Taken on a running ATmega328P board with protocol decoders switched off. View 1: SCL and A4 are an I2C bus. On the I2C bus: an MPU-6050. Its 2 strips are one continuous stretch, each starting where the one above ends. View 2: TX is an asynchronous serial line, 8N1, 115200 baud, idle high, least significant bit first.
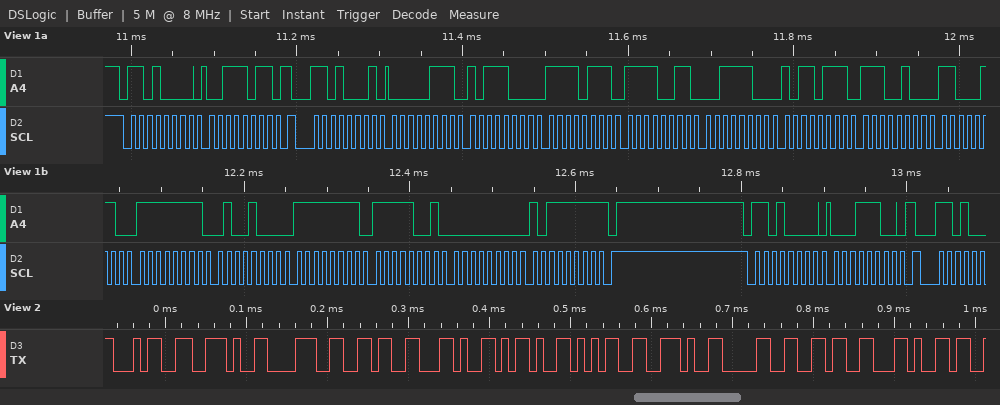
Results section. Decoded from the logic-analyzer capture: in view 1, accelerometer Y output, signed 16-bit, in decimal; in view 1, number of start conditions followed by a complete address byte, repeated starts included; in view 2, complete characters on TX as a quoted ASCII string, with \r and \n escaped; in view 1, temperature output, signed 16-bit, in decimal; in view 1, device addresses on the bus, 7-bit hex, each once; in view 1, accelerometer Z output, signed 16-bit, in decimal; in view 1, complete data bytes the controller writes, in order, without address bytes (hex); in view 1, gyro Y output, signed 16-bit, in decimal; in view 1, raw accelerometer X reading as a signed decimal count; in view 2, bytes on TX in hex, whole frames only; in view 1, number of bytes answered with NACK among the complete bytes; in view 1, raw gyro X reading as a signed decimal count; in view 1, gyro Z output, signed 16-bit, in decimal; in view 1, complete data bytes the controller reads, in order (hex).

-2061
3
"4.86,-5.06,"
-6970
0x68
15543
3B 1C
-7
1976
34 2E 38 36 2C 2D 35 2E 30 36 2C
1
-184
191
07 B8 F7 F3 3C B7 E4 C6 FF 48 FF F9 00 BF
